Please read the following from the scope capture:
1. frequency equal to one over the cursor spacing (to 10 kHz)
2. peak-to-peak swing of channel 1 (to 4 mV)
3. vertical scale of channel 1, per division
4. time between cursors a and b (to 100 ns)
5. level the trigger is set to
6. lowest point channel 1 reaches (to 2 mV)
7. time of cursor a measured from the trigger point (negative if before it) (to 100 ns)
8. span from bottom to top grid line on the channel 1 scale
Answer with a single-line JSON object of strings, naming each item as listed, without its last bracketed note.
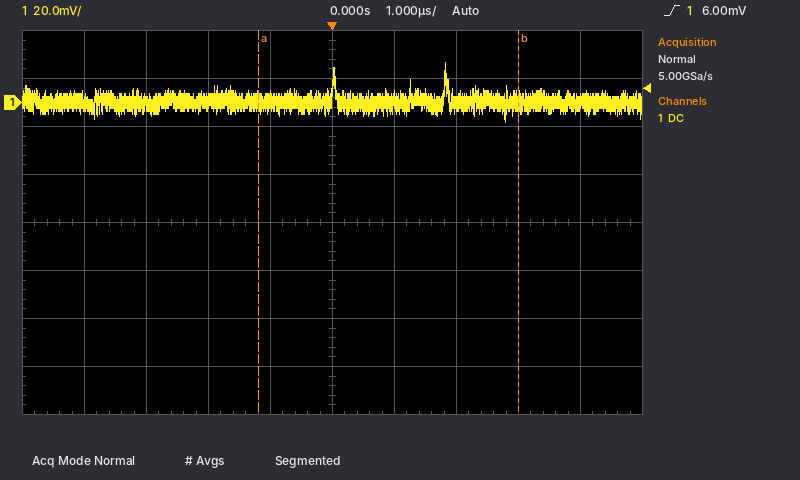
{"frequency equal to one over the cursor spacing": "240 kHz", "peak-to-peak swing of channel 1": "24 mV", "vertical scale of channel 1, per division": "20 mV", "time between cursors a and b": "4.2 µs", "level the trigger is set to": "6.00 mV", "lowest point channel 1 reaches": "-8 mV", "time of cursor a measured from the trigger point (negative if before it)": "-1.2 µs", "span from bottom to top grid line on the channel 1 scale": "160 mV"}
